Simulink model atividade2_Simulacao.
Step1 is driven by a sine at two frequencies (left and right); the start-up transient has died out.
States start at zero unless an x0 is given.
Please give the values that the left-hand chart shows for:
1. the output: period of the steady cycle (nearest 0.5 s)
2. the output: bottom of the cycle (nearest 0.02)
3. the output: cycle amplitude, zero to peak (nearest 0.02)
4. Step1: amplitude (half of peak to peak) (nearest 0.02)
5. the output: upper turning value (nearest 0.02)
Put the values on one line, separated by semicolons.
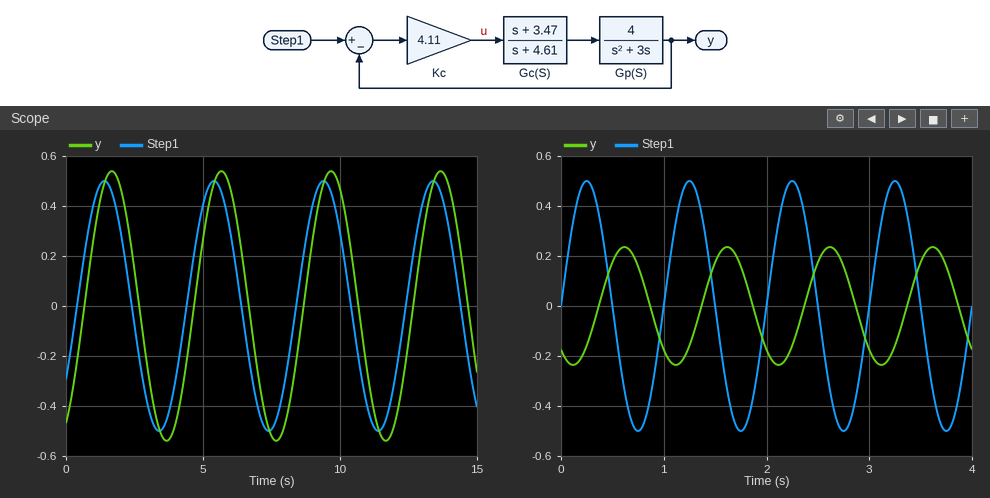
4.0 s; -0.54; 0.54; 0.50; 0.54
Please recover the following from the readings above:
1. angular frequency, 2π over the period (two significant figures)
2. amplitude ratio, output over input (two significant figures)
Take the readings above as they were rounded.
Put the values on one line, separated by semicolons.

1.6 rad/s; 1.1
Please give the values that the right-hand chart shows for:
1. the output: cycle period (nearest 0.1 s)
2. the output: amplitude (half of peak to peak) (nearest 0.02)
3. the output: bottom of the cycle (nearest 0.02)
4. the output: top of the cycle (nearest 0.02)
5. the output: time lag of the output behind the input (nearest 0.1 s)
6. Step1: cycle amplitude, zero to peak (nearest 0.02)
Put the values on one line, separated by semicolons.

1.0 s; 0.24; -0.24; 0.24; 0.4 s; 0.50
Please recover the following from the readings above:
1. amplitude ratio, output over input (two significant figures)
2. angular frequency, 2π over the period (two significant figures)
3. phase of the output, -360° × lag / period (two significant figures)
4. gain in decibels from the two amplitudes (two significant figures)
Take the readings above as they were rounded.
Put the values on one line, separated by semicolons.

0.48; 6.3 rad/s; -140°; -6.4 dB
